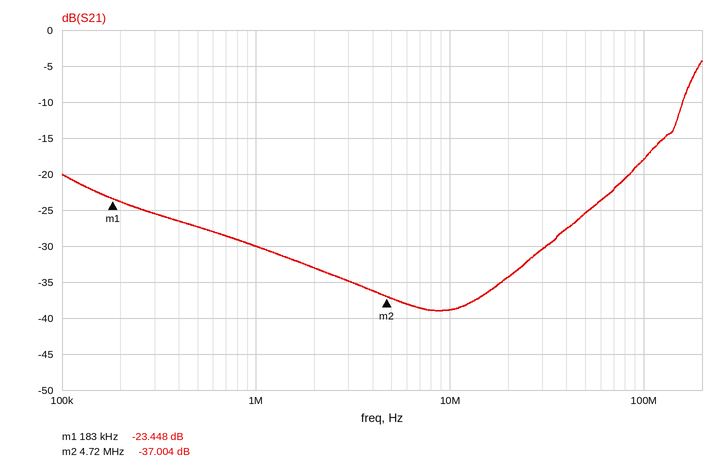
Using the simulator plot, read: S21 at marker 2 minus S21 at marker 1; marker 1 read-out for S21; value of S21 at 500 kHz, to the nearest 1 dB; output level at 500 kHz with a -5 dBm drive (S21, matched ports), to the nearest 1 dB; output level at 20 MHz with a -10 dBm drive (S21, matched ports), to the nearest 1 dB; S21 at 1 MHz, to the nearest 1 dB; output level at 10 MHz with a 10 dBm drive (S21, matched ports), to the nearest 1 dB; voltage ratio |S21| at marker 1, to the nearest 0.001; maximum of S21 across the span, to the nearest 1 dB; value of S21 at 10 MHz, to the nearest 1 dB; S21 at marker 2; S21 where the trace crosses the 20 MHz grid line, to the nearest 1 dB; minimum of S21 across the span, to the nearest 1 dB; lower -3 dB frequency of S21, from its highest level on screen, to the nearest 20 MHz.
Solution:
-13.556 dB
-23.448 dB
-27 dB
-32 dBm
-44 dBm
-30 dB
-29 dBm
0.067
-4 dB
-39 dB
-37.004 dB
-34 dB
-39 dB
180 MHz
